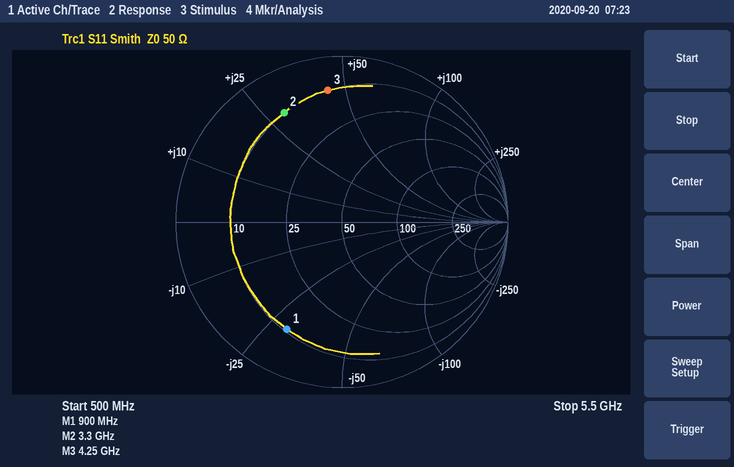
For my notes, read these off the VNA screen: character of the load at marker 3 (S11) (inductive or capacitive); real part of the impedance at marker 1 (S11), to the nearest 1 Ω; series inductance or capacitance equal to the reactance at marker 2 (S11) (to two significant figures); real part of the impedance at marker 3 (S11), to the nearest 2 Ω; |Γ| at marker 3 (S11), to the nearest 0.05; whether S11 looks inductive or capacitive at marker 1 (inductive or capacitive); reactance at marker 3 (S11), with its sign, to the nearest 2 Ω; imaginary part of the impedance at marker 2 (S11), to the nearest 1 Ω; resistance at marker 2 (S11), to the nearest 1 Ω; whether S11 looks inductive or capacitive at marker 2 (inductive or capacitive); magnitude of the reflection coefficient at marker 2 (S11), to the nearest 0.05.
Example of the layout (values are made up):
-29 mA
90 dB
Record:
inductive
11 Ω
1.4 nH
10 Ω
0.80
capacitive
+44 Ω
+29 Ω
10 Ω
inductive
0.75
